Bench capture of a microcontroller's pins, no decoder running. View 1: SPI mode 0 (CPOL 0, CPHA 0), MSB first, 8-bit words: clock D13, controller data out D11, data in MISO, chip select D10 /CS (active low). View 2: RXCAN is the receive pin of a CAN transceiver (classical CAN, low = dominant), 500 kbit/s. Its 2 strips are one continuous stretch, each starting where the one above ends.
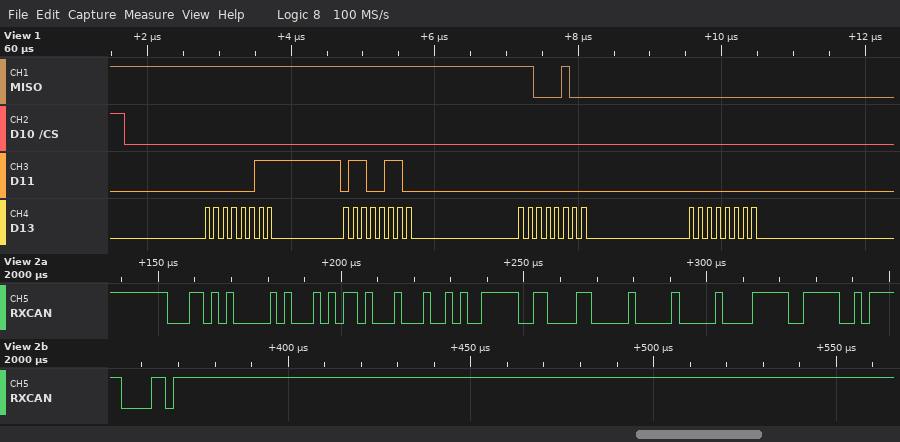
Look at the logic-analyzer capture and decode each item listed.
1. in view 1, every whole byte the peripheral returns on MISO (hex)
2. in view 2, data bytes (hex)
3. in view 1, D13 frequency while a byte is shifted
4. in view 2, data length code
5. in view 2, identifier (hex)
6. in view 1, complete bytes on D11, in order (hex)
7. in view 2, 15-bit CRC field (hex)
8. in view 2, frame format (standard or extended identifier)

FF FF C4 00
AD 11 29 F6 18 00 00 FB
8 MHz
8
0x1A8
03 66 00 00
0x75F1
standard
